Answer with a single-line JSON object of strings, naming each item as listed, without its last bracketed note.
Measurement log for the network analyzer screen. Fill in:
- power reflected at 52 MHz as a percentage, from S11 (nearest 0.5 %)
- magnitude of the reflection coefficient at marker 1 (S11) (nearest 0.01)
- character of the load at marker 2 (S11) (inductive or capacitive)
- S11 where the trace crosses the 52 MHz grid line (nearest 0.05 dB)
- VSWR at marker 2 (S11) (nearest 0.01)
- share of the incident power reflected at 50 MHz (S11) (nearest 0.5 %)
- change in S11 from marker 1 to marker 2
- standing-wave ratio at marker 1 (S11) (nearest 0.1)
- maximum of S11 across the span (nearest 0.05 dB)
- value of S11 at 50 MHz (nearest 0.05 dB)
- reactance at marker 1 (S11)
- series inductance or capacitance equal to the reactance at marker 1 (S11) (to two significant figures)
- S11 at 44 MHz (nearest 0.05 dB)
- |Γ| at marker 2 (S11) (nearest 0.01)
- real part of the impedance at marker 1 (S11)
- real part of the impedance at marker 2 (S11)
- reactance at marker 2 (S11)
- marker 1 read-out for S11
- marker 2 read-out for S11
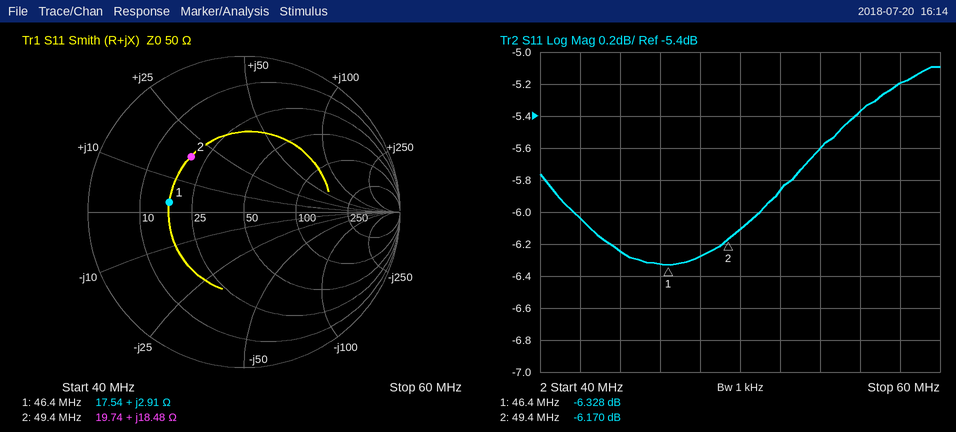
{"power reflected at 52 MHz as a percentage, from S11": "26.0 %", "magnitude of the reflection coefficient at marker 1 (S11)": "0.48", "character of the load at marker 2 (S11)": "inductive", "S11 where the trace crosses the 52 MHz grid line": "-5.85 dB", "VSWR at marker 2 (S11)": "2.93", "share of the incident power reflected at 50 MHz (S11)": "24.5 %", "change in S11 from marker 1 to marker 2": "0.158 dB", "standing-wave ratio at marker 1 (S11)": "2.9", "maximum of S11 across the span": "-5.10 dB", "value of S11 at 50 MHz": "-6.10 dB", "reactance at marker 1": "+2.91 Ω", "series inductance or capacitance equal to the reactance at marker 1 (S11)": "10.0 nH", "S11 at 44 MHz": "-6.25 dB", "|Γ| at marker 2 (S11)": "0.49", "real part of the impedance at marker 1": "17.54 Ω", "real part of the impedance at marker 2": "19.74 Ω", "reactance at marker 2": "+18.48 Ω", "marker 1 read-out for S11": "-6.328 dB", "marker 2 read-out for S11": "-6.170 dB"}
